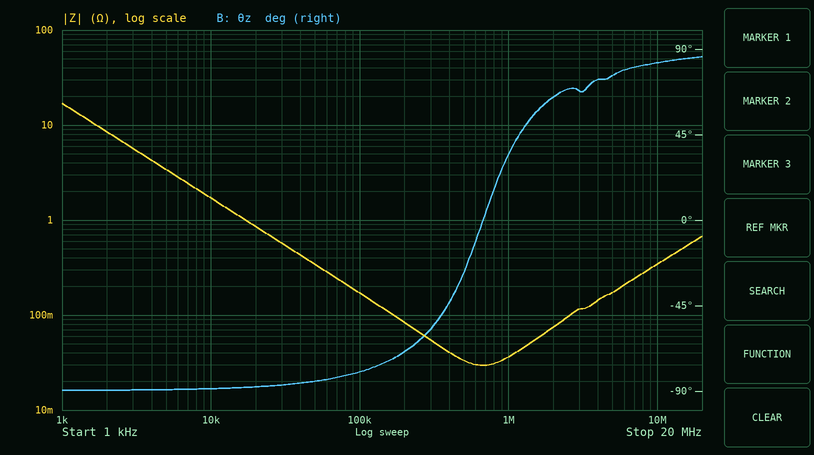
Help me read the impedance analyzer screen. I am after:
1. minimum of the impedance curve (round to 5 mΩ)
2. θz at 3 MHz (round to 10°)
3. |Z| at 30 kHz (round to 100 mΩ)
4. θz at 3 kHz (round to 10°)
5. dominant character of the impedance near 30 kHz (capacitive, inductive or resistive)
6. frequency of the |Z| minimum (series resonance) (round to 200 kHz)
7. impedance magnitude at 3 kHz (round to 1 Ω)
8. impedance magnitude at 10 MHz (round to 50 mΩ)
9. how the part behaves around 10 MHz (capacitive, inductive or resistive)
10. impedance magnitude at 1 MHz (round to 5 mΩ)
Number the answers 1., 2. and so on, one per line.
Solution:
1. 30 mΩ
2. 70°
3. 600 mΩ
4. -90°
5. capacitive
6. 600 kHz
7. 6 Ω
8. 350 mΩ
9. inductive
10. 35 mΩ
